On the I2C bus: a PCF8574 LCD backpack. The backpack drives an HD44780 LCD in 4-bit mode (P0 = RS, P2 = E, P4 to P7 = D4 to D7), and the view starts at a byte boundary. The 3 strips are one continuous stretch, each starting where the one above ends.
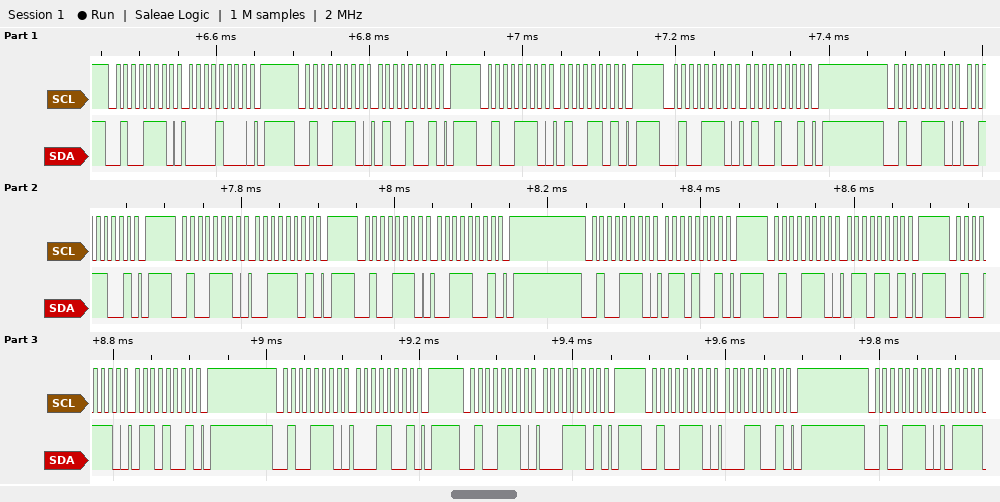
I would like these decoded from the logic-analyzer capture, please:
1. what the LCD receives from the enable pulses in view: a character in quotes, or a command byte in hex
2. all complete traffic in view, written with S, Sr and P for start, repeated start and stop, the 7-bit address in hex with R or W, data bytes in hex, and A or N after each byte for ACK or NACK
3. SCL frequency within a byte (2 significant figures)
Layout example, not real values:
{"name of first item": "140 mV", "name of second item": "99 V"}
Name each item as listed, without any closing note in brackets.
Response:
{"what the LCD receives from the enable pulses in view: a character in quotes, or a command byte in hex": "'C' 'a'", "all complete traffic in view, written with S, Sr and P for start, repeated start and stop, the 7-bit address in hex with R or W, data bytes in hex, and A or N after each byte for ACK or NACK": "S 27W A 08 A P S 27W A 49 A P S 27W A 4D A P S 27W A 49 A P S 27W A 39 A P S 27W A 3D A P S 27W A 39 A P S 27W A 69 A P S 27W A 6D A P S 27W A 69 A P S 27W A 19 A P S 27W A 1D A P S 27W A 19 A P S 27W A", "SCL frequency within a byte": "100 kHz"}
